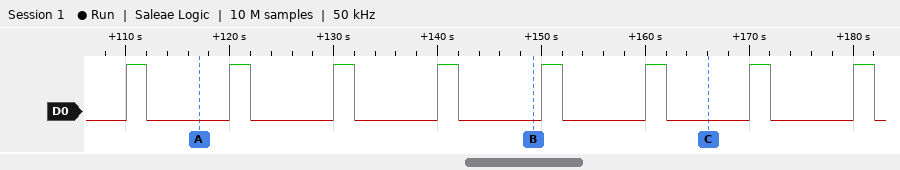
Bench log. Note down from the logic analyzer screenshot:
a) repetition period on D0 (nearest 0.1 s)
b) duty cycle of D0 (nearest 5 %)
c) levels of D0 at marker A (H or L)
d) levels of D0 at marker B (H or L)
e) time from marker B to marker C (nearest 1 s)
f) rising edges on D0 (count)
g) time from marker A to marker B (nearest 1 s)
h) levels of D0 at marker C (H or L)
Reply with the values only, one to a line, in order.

10 s
20 %
D0=L
D0=L
17 s
8
32 s
D0=L
